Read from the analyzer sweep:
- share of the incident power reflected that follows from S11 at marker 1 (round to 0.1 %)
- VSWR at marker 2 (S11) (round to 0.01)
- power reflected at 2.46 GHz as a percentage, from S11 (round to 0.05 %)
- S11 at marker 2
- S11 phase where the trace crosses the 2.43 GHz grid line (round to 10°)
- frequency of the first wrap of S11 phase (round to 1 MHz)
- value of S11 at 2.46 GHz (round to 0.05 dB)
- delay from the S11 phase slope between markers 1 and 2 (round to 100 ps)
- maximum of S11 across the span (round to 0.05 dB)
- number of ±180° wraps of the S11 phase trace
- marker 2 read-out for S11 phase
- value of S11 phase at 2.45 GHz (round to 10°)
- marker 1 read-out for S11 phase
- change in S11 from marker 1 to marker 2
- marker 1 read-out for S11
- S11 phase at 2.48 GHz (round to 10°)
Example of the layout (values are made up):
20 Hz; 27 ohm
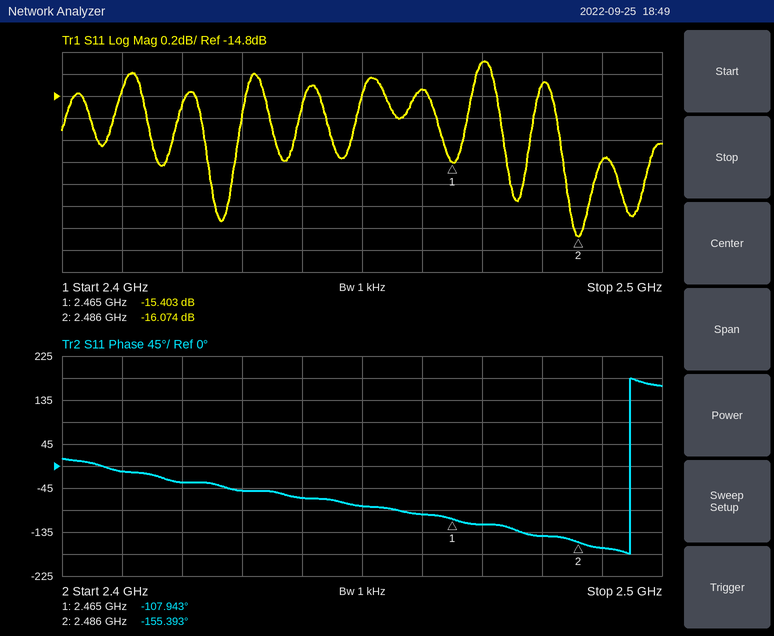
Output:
2.9 %; 1.37; 3.35 %; -16.074 dB; -50°; 2.495 GHz; -14.75 dB; 6.3 ns; -14.50 dB; 1; -155.393°; -80°; -107.943°; -0.671 dB; -15.403 dB; -140°
